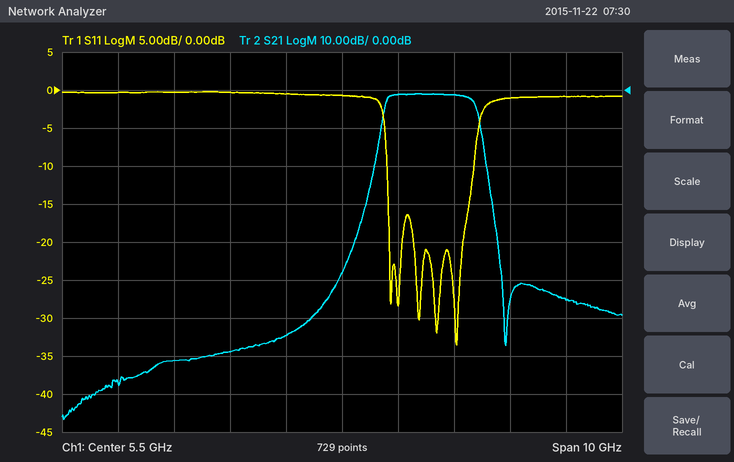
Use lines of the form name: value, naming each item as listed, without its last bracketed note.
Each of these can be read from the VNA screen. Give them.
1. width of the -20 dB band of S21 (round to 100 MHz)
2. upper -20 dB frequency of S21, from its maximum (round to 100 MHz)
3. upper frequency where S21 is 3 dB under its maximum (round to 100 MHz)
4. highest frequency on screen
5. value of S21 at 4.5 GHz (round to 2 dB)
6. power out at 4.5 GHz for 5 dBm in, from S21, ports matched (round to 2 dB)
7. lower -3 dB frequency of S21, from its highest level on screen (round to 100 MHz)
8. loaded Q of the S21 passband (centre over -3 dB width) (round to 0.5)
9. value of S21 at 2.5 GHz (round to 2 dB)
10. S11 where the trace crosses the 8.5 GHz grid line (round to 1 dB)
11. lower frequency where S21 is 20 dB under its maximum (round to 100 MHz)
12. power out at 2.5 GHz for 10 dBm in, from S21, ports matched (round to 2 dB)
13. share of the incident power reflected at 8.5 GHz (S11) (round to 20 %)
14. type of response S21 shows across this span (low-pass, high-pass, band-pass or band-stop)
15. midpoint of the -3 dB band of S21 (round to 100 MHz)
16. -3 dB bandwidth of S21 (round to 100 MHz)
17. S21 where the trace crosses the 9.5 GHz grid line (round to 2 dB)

width of the -20 dB band of S21: 2.0 GHz
upper -20 dB frequency of S21, from its maximum: 8.1 GHz
upper frequency where S21 is 3 dB under its maximum: 7.9 GHz
highest frequency on screen: 10.5 GHz
value of S21 at 4.5 GHz: -64 dB
power out at 4.5 GHz for 5 dBm in, from S21, ports matched: -60 dBm
lower -3 dB frequency of S21, from its highest level on screen: 6.3 GHz
loaded Q of the S21 passband (centre over -3 dB width): 4.5
value of S21 at 2.5 GHz: -72 dB
S11 where the trace crosses the 8.5 GHz grid line: -1 dB
lower frequency where S21 is 20 dB under its maximum: 6.1 GHz
power out at 2.5 GHz for 10 dBm in, from S21, ports matched: -62 dBm
share of the incident power reflected at 8.5 GHz (S11): 80 %
type of response S21 shows across this span: band-pass
midpoint of the -3 dB band of S21: 7.1 GHz
-3 dB bandwidth of S21: 1.6 GHz
S21 where the trace crosses the 9.5 GHz grid line: -56 dB
